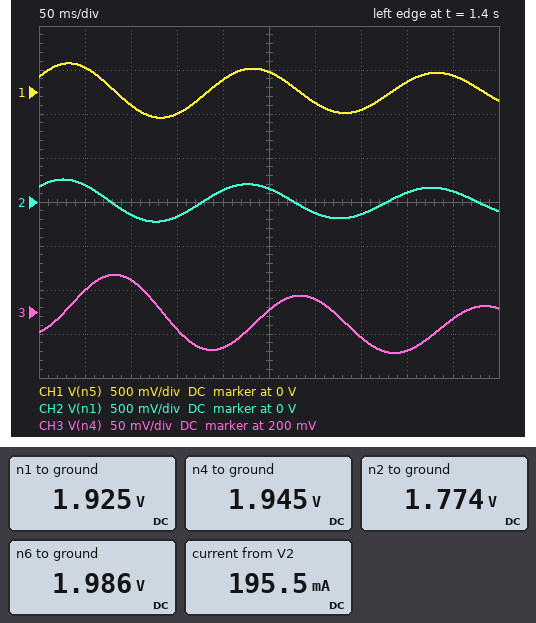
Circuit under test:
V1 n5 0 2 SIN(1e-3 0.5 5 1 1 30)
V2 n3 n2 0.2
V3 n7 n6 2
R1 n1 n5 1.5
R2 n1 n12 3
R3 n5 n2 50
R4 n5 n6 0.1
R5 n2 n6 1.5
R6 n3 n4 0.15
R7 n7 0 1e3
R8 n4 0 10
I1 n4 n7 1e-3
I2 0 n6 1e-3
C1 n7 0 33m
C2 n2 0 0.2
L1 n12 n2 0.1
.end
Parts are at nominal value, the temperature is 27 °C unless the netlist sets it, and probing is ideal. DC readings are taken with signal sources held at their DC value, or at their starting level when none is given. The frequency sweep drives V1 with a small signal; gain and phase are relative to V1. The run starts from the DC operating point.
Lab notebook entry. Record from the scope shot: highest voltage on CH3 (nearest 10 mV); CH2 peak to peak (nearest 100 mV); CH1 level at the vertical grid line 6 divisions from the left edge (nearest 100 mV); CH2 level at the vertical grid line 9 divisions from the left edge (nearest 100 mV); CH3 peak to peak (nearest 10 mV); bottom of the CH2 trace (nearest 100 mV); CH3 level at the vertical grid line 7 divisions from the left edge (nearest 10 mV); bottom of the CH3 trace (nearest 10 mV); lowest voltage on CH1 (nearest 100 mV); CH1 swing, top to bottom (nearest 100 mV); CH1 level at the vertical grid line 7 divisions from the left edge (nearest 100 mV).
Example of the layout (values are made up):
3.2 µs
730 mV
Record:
240 mV
500 mV
-100 mV
100 mV
90 mV
-200 mV
170 mV
150 mV
-300 mV
600 mV
-200 mV
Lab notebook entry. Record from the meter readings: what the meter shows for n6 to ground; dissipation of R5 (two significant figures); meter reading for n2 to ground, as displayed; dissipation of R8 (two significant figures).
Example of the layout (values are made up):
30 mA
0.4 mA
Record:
1.986 V
30 mW
1.774 V
380 mW
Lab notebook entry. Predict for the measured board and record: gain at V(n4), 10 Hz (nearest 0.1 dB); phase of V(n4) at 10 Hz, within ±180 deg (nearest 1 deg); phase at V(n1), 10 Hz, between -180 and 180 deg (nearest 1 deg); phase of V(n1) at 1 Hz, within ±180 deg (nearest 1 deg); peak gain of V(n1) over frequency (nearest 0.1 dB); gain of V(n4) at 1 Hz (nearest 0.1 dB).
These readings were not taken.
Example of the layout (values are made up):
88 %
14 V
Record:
-24.8 dB
-104 deg
10 deg
-9 deg
0 dB
-5.3 dB
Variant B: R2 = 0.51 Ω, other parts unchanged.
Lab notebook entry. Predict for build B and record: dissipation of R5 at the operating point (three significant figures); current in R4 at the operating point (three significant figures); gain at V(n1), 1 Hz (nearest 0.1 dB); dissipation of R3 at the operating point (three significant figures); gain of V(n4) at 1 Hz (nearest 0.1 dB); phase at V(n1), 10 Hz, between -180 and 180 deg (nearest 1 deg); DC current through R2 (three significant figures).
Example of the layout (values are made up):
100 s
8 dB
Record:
18.0 mW
112 mA
-5.2 dB
616 µW
-3.5 dB
13 deg
87.3 mA
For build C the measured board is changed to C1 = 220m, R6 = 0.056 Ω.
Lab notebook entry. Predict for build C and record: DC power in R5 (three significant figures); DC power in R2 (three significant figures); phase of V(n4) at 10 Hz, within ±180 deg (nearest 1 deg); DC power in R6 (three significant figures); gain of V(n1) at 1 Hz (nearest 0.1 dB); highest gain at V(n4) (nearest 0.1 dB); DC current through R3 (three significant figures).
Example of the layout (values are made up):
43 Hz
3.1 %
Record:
30.3 mW
7.67 mW
-137 deg
2.18 mW
-2.5 dB
-1.0 dB
4.55 mA
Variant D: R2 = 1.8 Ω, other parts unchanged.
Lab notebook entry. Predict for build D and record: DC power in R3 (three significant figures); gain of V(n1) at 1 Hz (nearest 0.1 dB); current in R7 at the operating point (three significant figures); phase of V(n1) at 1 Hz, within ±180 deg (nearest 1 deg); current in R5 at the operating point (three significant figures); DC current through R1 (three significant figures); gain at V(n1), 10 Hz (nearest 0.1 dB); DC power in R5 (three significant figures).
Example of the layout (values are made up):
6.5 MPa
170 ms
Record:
867 µW
-3.2 dB
3.99 mA
-13 deg
130 mA
63.1 mA
-0.8 dB
25.3 mW
